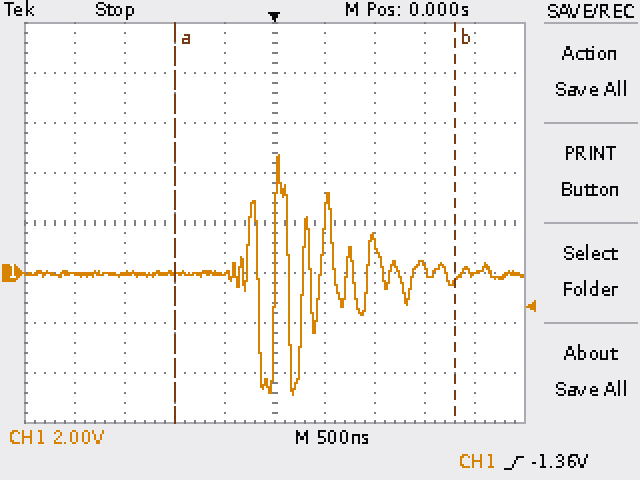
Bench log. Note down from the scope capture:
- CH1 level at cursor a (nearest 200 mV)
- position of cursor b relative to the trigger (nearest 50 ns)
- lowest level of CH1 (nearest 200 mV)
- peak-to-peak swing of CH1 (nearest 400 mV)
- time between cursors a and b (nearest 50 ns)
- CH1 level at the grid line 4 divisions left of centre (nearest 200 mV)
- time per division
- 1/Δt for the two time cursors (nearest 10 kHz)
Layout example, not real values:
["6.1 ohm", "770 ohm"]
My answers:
["0.0 V", "+1.80 µs", "-4.8 V", "9.6 V", "2.80 µs", "0.0 V", "500 ns", "360 kHz"]
